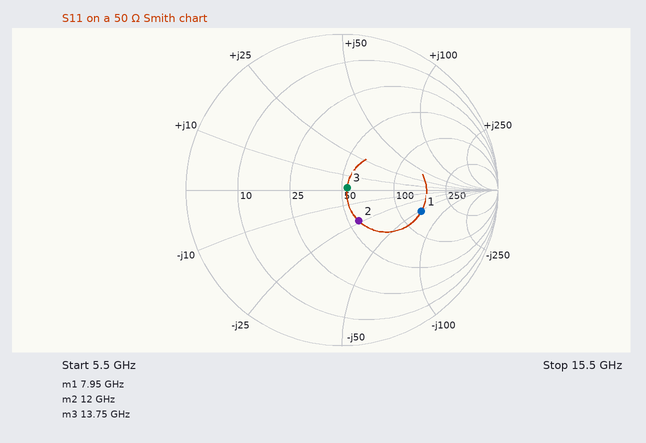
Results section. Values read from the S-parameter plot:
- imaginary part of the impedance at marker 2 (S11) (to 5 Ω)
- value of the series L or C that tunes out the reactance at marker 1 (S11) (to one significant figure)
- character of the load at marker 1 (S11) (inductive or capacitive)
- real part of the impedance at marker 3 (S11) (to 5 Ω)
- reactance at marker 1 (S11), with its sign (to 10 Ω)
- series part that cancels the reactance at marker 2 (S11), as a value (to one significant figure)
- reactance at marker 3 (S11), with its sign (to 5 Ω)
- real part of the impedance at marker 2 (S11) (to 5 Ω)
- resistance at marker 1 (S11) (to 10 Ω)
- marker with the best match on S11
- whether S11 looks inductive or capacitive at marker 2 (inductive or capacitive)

-25 Ω
1 nH
capacitive
55 Ω
-50 Ω
300 pH
0 Ω
55 Ω
140 Ω
marker 3
capacitive
